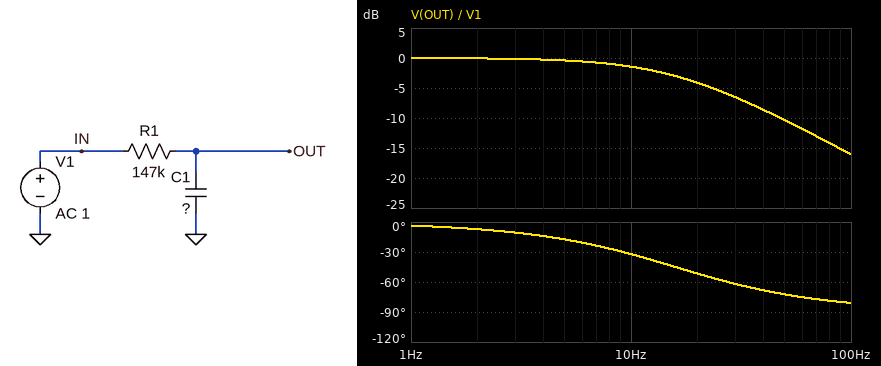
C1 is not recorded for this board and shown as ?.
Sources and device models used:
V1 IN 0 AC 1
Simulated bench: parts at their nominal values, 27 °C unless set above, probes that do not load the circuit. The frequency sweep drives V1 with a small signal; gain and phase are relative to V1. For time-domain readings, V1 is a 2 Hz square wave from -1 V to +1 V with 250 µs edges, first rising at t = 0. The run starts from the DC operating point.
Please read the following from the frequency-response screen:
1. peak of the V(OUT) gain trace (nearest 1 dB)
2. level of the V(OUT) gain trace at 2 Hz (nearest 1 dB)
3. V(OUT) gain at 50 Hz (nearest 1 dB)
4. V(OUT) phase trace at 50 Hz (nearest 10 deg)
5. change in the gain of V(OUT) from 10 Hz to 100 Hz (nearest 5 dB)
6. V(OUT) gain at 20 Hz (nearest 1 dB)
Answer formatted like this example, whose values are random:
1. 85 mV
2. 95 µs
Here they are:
1. 0 dB
2. 0 dB
3. -10 dB
4. -70 deg
5. -15 dB
6. -4 dB
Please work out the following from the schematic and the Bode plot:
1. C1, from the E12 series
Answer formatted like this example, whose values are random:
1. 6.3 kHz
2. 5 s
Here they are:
1. 68 nF
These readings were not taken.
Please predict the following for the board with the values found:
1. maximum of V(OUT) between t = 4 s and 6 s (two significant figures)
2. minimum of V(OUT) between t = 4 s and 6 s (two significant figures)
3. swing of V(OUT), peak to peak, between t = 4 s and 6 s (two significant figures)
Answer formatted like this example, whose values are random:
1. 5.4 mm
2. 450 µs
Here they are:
1. 1.0 V
2. -1.0 V
3. 2.0 V
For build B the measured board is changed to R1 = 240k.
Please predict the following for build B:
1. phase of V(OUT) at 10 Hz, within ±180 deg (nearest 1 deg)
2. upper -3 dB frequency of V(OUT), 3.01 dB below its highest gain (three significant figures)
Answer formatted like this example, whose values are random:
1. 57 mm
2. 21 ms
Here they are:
1. -46 deg
2. 9.75 Hz
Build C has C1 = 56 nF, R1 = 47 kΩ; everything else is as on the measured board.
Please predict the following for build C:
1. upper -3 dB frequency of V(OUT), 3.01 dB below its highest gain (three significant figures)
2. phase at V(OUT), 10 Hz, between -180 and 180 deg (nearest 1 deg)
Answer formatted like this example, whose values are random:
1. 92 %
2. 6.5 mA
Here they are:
1. 60.5 Hz
2. -9 deg
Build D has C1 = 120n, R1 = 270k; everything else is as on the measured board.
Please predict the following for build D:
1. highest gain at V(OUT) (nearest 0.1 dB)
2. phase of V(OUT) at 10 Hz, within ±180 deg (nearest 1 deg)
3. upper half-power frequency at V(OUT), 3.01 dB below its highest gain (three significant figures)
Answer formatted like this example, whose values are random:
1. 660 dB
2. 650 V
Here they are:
1. 0 dB
2. -64 deg
3. 4.91 Hz
